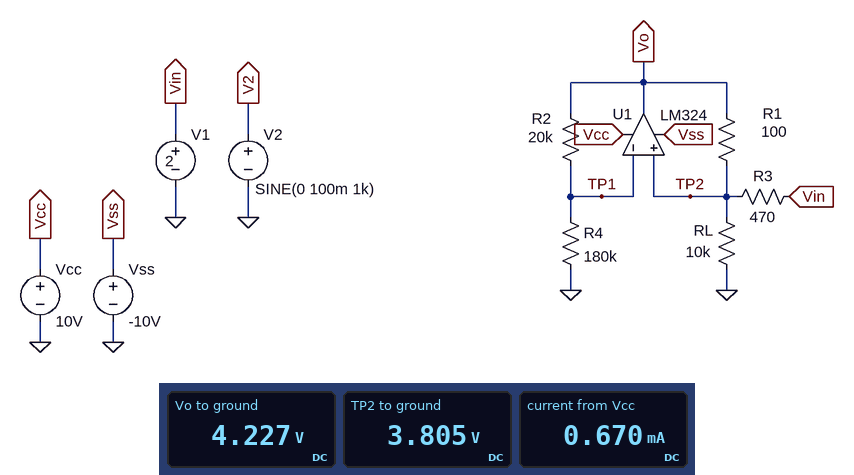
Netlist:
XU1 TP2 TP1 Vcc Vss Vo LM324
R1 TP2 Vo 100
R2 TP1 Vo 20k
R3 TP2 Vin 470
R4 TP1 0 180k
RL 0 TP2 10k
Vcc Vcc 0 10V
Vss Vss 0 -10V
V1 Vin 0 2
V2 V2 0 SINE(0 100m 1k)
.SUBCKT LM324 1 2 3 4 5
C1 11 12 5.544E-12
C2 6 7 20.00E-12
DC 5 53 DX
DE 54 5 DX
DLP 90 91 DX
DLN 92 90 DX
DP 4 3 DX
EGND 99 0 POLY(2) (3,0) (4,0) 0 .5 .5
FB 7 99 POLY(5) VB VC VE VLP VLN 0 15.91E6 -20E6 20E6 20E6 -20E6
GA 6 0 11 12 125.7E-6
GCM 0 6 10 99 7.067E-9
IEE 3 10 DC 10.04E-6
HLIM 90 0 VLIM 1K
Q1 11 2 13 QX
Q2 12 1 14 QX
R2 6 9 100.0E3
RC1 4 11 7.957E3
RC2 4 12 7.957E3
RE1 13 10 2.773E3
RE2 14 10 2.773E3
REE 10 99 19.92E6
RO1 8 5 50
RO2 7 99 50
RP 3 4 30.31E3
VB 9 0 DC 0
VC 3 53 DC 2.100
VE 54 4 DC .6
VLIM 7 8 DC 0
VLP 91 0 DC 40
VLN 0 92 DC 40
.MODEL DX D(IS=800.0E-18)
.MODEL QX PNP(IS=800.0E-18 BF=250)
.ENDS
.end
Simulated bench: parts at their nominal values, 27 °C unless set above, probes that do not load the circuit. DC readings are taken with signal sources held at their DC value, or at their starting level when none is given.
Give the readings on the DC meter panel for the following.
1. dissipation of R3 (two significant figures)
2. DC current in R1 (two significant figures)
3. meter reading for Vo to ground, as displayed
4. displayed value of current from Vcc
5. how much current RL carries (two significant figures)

6.9 mW
4.2 mA
4.227 V
0.670 mA
380 µA
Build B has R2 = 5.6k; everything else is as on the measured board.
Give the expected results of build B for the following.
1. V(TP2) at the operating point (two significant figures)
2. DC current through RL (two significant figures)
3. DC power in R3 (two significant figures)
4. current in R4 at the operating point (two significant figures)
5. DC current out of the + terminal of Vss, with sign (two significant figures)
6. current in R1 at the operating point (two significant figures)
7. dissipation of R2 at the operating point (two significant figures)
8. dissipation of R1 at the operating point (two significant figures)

2.2 V
220 µA
100 µW
12 µA
-670 µA
690 µA
850 nW
47 µW
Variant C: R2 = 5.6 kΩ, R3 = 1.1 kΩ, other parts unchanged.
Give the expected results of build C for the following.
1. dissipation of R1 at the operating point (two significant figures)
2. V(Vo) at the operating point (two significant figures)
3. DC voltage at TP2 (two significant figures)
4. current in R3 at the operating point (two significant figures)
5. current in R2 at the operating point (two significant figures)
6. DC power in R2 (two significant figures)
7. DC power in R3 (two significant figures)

65 µW
2.7 V
2.6 V
550 µA
14 µA
1.2 µW
330 µW
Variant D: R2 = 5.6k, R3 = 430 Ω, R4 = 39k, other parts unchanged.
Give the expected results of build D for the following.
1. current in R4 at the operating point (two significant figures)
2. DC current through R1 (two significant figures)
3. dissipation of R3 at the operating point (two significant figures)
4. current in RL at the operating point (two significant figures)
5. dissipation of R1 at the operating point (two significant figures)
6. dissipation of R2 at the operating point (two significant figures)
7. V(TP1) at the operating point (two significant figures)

120 µA
6.7 mA
17 mW
470 µA
4.5 mW
81 µW
4.7 V
